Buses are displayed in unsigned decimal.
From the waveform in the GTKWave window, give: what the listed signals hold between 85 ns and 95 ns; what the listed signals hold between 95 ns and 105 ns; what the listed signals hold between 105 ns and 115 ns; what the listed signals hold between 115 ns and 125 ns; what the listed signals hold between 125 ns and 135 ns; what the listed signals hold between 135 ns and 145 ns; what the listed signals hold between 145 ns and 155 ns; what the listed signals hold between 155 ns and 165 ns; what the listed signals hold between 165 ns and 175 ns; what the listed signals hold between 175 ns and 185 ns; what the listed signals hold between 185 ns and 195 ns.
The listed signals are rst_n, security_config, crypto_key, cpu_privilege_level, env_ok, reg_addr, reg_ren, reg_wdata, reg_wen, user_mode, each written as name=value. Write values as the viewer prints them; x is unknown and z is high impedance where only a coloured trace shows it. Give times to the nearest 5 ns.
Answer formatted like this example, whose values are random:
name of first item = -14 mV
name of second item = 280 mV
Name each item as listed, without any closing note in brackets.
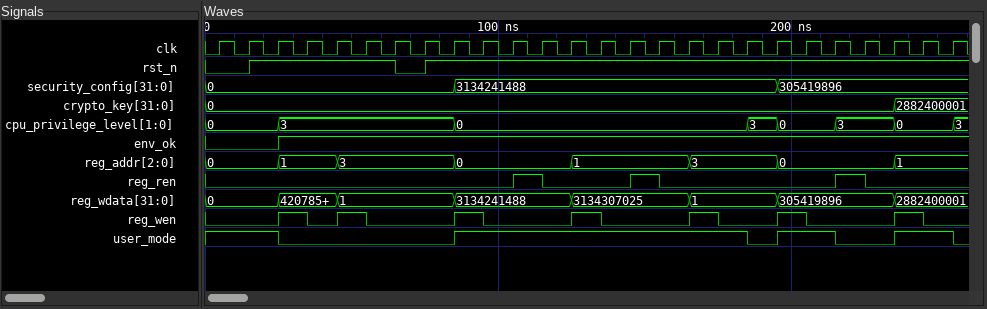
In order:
what the listed signals hold between 85 ns and 95 ns = rst_n=1, security_config=3134241488, crypto_key=0, cpu_privilege_level=0, env_ok=1, reg_addr=0, reg_ren=0, reg_wdata=3134241488, reg_wen=1, user_mode=1
what the listed signals hold between 95 ns and 105 ns = rst_n=1, security_config=3134241488, crypto_key=0, cpu_privilege_level=0, env_ok=1, reg_addr=0, reg_ren=0, reg_wdata=3134241488, reg_wen=0, user_mode=1
what the listed signals hold between 105 ns and 115 ns = rst_n=1, security_config=3134241488, crypto_key=0, cpu_privilege_level=0, env_ok=1, reg_addr=0, reg_ren=1, reg_wdata=3134241488, reg_wen=0, user_mode=1
what the listed signals hold between 115 ns and 125 ns = rst_n=1, security_config=3134241488, crypto_key=0, cpu_privilege_level=0, env_ok=1, reg_addr=0, reg_ren=0, reg_wdata=3134241488, reg_wen=0, user_mode=1
what the listed signals hold between 125 ns and 135 ns = rst_n=1, security_config=3134241488, crypto_key=0, cpu_privilege_level=0, env_ok=1, reg_addr=1, reg_ren=0, reg_wdata=3134307025, reg_wen=1, user_mode=1
what the listed signals hold between 135 ns and 145 ns = rst_n=1, security_config=3134241488, crypto_key=0, cpu_privilege_level=0, env_ok=1, reg_addr=1, reg_ren=0, reg_wdata=3134307025, reg_wen=0, user_mode=1
what the listed signals hold between 145 ns and 155 ns = rst_n=1, security_config=3134241488, crypto_key=0, cpu_privilege_level=0, env_ok=1, reg_addr=1, reg_ren=1, reg_wdata=3134307025, reg_wen=0, user_mode=1
what the listed signals hold between 155 ns and 165 ns = rst_n=1, security_config=3134241488, crypto_key=0, cpu_privilege_level=0, env_ok=1, reg_addr=1, reg_ren=0, reg_wdata=3134307025, reg_wen=0, user_mode=1
what the listed signals hold between 165 ns and 175 ns = rst_n=1, security_config=3134241488, crypto_key=0, cpu_privilege_level=0, env_ok=1, reg_addr=3, reg_ren=0, reg_wdata=1, reg_wen=1, user_mode=1
what the listed signals hold between 175 ns and 185 ns = rst_n=1, security_config=3134241488, crypto_key=0, cpu_privilege_level=0, env_ok=1, reg_addr=3, reg_ren=0, reg_wdata=1, reg_wen=0, user_mode=1
what the listed signals hold between 185 ns and 195 ns = rst_n=1, security_config=3134241488, crypto_key=0, cpu_privilege_level=3, env_ok=1, reg_addr=3, reg_ren=0, reg_wdata=1, reg_wen=0, user_mode=0
